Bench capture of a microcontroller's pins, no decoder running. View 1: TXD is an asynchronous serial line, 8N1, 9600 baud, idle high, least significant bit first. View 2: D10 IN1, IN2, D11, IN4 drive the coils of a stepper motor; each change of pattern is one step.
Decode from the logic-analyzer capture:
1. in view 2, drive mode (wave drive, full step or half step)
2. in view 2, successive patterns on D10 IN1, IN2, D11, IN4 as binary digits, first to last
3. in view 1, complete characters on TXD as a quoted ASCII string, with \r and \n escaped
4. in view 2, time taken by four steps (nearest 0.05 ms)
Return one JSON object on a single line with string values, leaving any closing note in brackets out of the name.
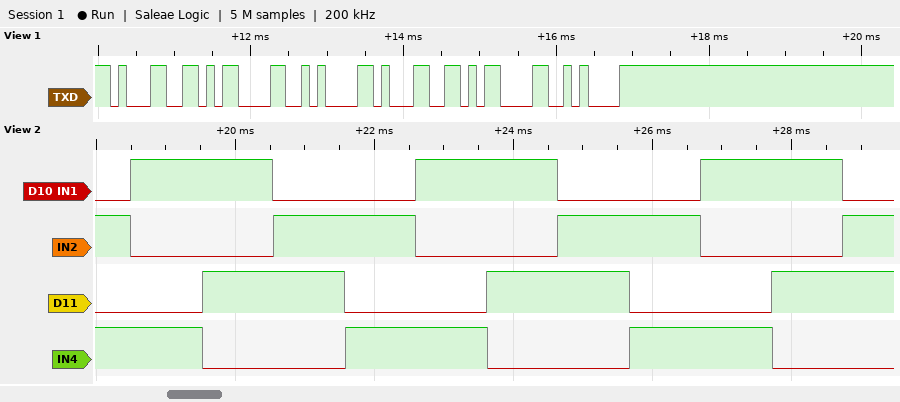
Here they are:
{"in view 2, drive mode": "full step", "in view 2, successive patterns on D10 IN1, IN2, D11, IN4 as binary digits, first to last": "0101 1001 1010 0110 0101 1001 1010 0110 0101 1001 1010 0110", "in view 1, complete characters on TXD as a quoted ASCII string, with \\r and \\n escaped": "\"1\\r\\n1\\r\\n\"", "in view 2, time taken by four steps": "4.10 ms"}
